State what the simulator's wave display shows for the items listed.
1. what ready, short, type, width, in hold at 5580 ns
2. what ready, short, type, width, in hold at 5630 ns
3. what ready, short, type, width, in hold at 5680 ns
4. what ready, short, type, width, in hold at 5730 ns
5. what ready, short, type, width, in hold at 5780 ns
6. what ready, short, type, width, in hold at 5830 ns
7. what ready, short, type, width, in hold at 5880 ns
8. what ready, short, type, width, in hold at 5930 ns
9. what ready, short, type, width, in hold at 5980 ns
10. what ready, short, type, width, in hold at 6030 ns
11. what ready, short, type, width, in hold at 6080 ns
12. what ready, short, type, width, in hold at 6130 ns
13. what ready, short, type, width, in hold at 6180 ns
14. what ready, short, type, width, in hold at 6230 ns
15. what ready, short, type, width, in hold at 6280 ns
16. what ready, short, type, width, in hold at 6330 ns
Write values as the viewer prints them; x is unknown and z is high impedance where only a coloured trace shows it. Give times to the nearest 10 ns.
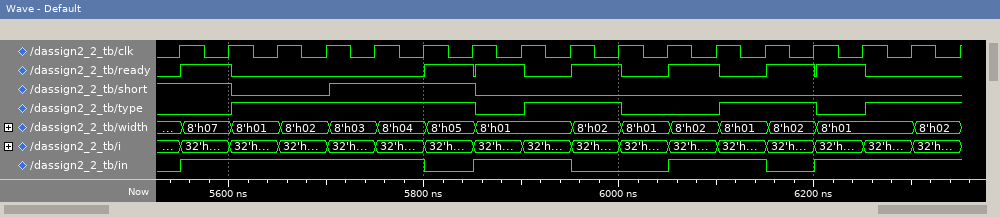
ready=1, short=1, type=0, width=8'h07, in=1
ready=0, short=0, type=1, width=8'h01, in=1
ready=0, short=0, type=1, width=8'h02, in=1
ready=0, short=1, type=1, width=8'h03, in=1
ready=0, short=1, type=1, width=8'h04, in=1
ready=1, short=1, type=1, width=8'h05, in=0
ready=1, short=0, type=0, width=8'h01, in=1
ready=0, short=0, type=1, width=8'h01, in=1
ready=1, short=0, type=1, width=8'h02, in=0
ready=0, short=0, type=0, width=8'h01, in=0
ready=1, short=0, type=0, width=8'h02, in=1
ready=0, short=0, type=1, width=8'h01, in=1
ready=1, short=0, type=1, width=8'h02, in=0
ready=1, short=0, type=0, width=8'h01, in=1
ready=0, short=0, type=1, width=8'h01, in=1
ready=0, short=0, type=1, width=8'h02, in=1
